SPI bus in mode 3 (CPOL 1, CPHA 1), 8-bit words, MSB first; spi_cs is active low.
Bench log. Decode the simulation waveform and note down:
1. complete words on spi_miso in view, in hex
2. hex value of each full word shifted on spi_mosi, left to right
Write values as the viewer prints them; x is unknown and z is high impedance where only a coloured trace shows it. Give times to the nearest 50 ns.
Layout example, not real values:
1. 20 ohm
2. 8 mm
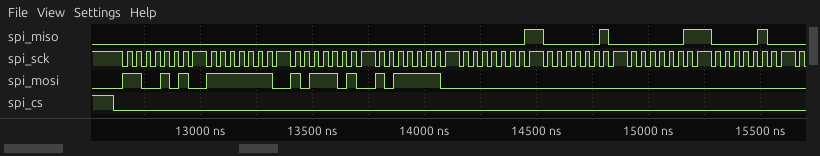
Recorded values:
1. 00, 00, 00, 00, 01, 02, 03, 04
2. CA, FE, BA, BE, 00, 00, 00, 00
